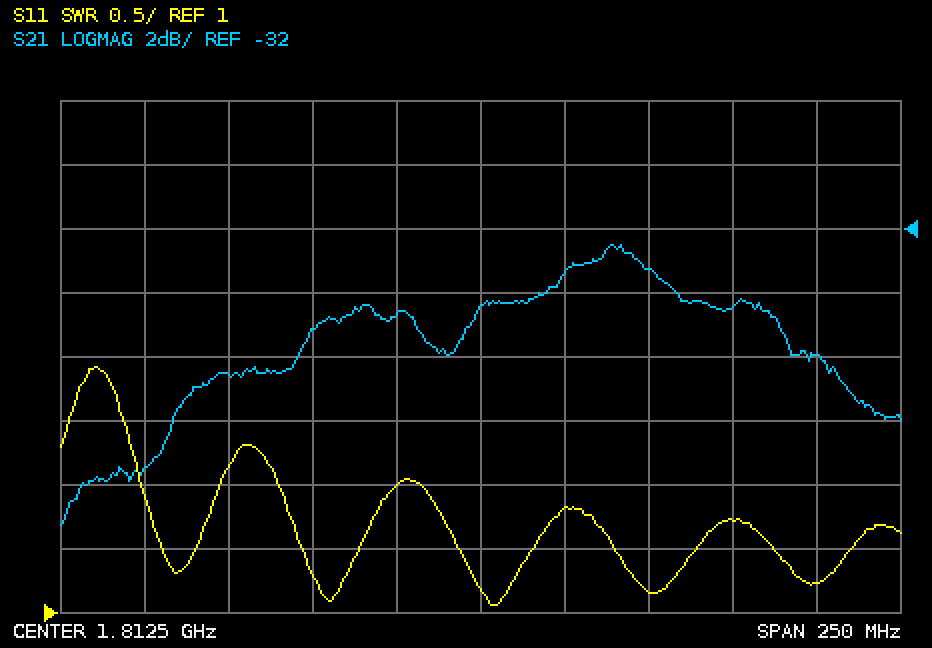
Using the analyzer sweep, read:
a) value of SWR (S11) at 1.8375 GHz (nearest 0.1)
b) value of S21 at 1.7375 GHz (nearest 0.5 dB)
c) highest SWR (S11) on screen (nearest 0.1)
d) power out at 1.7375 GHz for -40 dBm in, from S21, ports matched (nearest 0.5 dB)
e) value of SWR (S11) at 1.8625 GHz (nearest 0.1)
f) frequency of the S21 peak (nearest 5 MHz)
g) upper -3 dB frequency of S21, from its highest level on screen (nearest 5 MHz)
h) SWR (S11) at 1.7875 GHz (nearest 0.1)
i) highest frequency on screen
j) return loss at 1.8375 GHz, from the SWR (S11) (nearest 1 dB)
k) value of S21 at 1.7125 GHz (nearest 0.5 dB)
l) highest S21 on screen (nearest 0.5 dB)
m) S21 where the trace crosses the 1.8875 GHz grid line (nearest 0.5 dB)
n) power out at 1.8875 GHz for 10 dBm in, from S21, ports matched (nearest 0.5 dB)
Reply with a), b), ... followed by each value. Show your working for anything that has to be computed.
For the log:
a) 1.8
b) -36.5 dB
c) 2.9
d) -40 dBm + (-36.5 dB) = -76.5 dBm
e) 1.2
f) 1.850 GHz
g) 1.905 GHz
h) 2.0
i) 1.9375 GHz
j) −20 log10((1.8 − 1)/(1.8 + 1)) ≈ 11 dB
k) -39.5 dB
l) -32.5 dB
m) -34.5 dB
n) 10 dBm + (-34.5 dB) = -24.5 dBm
